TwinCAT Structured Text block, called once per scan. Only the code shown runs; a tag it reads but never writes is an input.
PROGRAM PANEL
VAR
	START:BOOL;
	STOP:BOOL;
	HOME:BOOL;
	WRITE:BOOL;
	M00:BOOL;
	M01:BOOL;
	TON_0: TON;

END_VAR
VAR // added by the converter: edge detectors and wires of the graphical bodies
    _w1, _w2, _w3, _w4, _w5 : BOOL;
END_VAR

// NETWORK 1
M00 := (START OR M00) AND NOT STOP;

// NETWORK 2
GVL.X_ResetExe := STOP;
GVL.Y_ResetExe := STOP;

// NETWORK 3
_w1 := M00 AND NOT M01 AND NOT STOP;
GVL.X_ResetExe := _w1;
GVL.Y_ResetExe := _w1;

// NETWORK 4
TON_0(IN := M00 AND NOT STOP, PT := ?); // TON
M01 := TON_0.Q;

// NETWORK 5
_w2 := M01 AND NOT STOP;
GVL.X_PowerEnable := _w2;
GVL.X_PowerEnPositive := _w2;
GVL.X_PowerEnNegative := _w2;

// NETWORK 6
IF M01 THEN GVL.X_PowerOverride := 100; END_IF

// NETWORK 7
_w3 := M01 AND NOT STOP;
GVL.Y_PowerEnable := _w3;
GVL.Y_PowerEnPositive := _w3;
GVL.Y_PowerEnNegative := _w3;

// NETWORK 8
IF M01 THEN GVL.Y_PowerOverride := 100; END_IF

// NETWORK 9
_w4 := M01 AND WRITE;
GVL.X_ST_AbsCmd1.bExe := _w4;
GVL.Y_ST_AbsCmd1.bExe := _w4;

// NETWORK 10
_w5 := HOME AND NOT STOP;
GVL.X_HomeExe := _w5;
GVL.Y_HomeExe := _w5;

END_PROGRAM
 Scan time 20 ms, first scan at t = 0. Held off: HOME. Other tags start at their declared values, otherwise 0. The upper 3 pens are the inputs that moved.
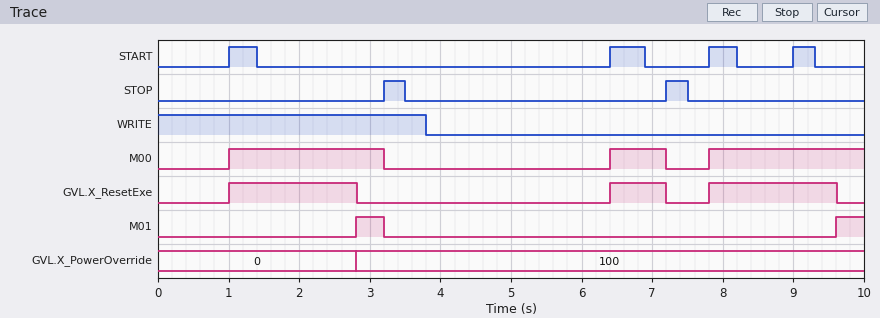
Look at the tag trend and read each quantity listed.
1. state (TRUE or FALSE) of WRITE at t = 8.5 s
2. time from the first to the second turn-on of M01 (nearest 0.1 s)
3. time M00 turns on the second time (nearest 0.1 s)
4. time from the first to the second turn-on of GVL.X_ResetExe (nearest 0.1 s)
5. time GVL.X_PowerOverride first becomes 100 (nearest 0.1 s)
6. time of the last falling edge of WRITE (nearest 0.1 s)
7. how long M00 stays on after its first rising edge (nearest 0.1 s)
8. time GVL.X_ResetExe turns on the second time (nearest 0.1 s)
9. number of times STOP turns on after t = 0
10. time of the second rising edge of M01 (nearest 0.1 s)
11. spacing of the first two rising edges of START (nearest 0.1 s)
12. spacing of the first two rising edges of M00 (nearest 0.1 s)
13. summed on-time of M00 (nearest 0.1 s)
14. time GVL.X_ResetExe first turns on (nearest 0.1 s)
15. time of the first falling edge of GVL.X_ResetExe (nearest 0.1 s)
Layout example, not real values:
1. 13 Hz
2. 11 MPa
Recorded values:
1. FALSE
2. 6.8 s
3. 6.4 s
4. 5.4 s
5. 2.8 s
6. 3.8 s
7. 2.2 s
8. 6.4 s
9. 2
10. 9.6 s
11. 5.4 s
12. 5.4 s
13. 5.2 s
14. 1.0 s
15. 2.8 s
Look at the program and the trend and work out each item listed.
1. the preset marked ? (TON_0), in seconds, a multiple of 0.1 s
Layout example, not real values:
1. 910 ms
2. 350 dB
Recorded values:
1. 1.8 s
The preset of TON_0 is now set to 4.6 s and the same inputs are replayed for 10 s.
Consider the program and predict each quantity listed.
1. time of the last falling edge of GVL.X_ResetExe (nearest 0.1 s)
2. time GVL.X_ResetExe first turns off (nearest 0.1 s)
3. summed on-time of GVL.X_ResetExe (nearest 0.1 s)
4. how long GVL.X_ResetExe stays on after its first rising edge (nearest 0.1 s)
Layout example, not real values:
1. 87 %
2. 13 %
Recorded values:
1. 7.2 s
2. 3.2 s
3. 5.2 s
4. 2.2 s
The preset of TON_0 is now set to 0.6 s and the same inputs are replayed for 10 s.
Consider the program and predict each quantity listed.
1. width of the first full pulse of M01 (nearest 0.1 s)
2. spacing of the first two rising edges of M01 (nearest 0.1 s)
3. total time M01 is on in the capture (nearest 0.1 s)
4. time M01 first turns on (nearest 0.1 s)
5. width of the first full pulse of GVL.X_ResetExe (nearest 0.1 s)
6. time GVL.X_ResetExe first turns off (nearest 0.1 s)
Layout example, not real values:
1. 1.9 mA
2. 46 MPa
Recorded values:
1. 1.6 s
2. 5.4 s
3. 3.4 s
4. 1.6 s
5. 0.6 s
6. 1.6 s
